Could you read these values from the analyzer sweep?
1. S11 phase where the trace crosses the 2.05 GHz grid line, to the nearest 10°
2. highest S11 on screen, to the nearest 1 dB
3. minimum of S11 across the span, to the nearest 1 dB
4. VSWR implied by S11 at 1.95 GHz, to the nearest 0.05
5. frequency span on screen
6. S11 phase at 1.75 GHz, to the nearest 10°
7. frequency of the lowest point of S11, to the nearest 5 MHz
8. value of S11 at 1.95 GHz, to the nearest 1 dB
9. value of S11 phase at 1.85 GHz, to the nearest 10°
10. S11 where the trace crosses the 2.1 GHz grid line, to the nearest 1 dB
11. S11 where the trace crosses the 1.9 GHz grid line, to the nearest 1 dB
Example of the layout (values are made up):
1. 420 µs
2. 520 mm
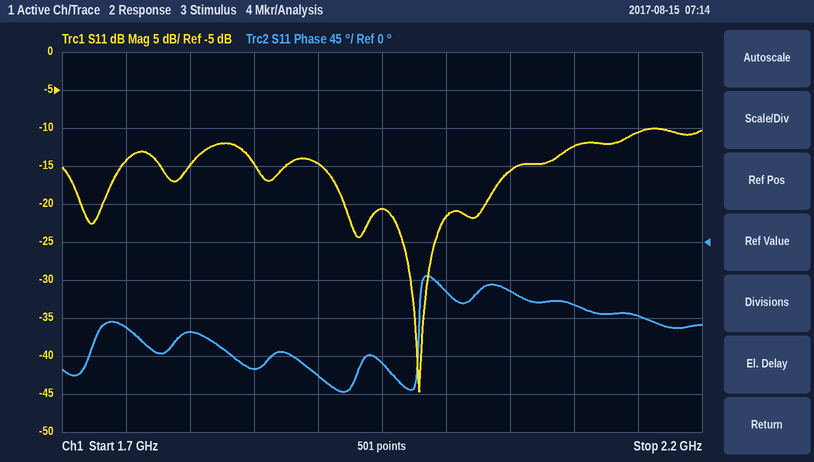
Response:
1. -60°
2. -10 dB
3. -45 dB
4. 1.20
5. 500 MHz
6. -100°
7. 1.980 GHz
8. -21 dB
9. -150°
10. -12 dB
11. -15 dB
